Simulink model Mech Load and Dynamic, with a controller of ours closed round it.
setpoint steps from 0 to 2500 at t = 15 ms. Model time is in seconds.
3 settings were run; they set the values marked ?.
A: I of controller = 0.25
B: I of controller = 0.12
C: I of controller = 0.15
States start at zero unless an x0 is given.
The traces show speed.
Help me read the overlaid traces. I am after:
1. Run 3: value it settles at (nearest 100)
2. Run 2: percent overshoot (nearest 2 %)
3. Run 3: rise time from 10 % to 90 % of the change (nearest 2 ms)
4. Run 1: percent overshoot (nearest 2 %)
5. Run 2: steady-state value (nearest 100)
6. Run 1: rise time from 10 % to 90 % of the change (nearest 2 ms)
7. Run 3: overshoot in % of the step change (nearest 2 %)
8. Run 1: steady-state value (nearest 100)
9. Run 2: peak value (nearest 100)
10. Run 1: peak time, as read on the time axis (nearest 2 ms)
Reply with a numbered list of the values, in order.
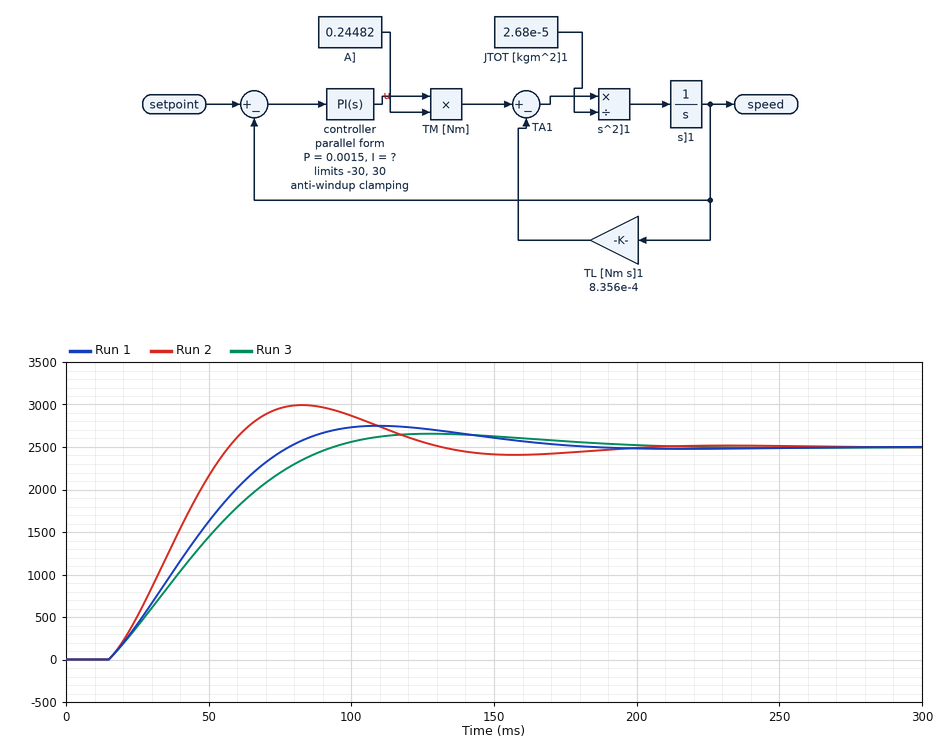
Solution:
1. 2500
2. 20 %
3. 56 ms
4. 10 %
5. 2500
6. 46 ms
7. 6 %
8. 2500
9. 3000
10. 110 ms
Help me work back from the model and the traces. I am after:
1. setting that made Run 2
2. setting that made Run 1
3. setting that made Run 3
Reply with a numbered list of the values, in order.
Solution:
1. A
2. C
3. B
